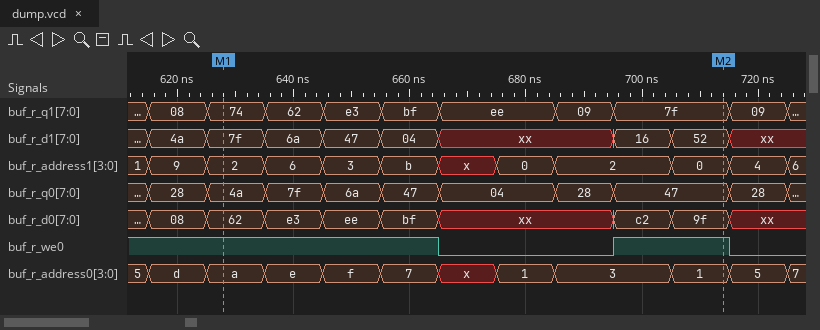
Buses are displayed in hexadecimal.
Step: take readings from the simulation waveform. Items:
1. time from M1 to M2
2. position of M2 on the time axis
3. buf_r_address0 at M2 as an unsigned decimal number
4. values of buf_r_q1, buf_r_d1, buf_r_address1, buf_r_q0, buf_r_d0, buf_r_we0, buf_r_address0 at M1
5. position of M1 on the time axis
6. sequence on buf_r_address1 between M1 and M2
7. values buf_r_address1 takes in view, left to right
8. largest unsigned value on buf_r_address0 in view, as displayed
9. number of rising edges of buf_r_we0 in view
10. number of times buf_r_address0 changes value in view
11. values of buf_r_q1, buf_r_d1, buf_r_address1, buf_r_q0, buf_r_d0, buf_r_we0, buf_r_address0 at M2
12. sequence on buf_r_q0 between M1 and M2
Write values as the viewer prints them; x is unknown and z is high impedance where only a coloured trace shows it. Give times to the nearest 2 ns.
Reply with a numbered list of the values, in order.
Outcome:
1. 86 ns
2. 714 ns
3. 1
4. buf_r_q1=74, buf_r_d1=7f, buf_r_address1=2, buf_r_q0=4a, buf_r_d0=62, buf_r_we0=1, buf_r_address0=a
5. 628 ns
6. 2, 6, 3, b, x, 0, 2, 0
7. 1, 9, 2, 6, 3, b, x, 0, 2, 0, 4, 6
8. f
9. 1
10. 11
11. buf_r_q1=7f, buf_r_d1=52, buf_r_address1=0, buf_r_q0=47, buf_r_d0=9f, buf_r_we0=1, buf_r_address0=1
12. 4a, 7f, 6a, 47, 04, 28, 47
